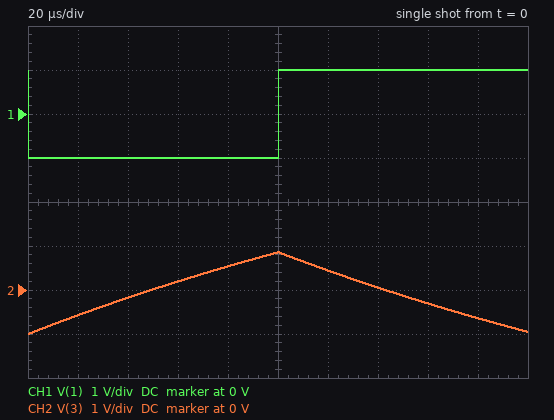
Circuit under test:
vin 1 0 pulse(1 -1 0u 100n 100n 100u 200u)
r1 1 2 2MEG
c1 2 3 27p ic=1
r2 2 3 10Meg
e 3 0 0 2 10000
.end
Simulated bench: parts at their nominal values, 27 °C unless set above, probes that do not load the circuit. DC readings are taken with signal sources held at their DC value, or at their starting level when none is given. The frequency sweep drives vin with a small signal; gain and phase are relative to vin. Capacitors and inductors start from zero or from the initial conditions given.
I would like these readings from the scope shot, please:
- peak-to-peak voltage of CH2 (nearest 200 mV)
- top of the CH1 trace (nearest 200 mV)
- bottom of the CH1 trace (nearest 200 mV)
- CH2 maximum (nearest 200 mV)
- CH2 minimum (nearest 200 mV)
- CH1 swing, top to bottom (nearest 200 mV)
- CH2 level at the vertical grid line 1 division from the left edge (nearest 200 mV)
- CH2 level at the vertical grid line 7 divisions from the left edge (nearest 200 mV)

1.8 V
1.0 V
-1.0 V
800 mV
-1.0 V
2.0 V
-600 mV
0 V
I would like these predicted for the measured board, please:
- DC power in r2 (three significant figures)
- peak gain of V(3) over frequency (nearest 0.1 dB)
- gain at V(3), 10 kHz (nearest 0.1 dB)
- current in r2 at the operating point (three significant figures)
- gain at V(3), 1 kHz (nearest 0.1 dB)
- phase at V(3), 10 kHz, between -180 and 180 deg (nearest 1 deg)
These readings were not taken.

2.50 µW
14.0 dB
-10.6 dB
500 nA
8.1 dB
93 deg
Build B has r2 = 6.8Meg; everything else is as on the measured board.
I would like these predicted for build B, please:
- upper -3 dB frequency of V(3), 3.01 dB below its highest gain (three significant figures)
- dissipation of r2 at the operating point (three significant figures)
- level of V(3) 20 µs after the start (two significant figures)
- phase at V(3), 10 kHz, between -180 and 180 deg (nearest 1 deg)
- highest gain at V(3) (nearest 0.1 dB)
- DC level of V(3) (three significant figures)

867 Hz
1.70 µW
-550 mV
95 deg
10.6 dB
-3.40 V
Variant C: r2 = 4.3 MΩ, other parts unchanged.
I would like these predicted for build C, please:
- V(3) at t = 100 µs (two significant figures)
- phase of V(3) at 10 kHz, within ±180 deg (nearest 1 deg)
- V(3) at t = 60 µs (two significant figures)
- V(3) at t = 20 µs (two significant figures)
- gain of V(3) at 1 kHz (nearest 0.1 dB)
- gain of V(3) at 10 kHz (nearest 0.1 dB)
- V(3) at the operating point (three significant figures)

820 mV
98 deg
270 mV
-500 mV
4.8 dB
-10.7 dB
-2.15 V
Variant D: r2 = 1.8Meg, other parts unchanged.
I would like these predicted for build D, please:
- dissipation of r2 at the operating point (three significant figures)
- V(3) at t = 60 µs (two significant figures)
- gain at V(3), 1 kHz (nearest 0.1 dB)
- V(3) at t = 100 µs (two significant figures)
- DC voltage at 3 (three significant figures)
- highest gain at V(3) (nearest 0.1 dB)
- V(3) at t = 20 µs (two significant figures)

450 nW
350 mV
-1.3 dB
660 mV
-900 mV
-0.9 dB
-360 mV
